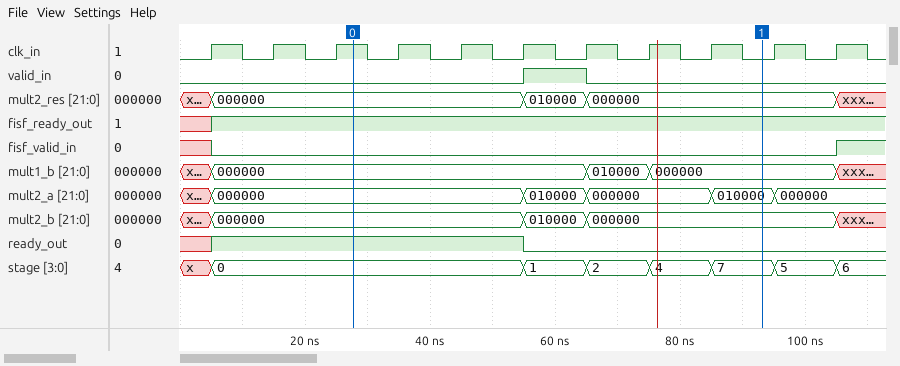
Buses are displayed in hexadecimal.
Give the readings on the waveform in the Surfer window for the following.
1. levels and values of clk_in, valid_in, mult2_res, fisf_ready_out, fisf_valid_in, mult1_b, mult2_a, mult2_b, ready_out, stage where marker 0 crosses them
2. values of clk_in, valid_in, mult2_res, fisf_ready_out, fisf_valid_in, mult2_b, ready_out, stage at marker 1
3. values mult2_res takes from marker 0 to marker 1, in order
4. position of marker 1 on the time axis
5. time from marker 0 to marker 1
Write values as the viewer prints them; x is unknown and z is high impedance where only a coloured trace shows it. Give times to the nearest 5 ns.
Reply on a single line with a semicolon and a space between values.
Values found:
clk_in=1, valid_in=0, mult2_res=000000, fisf_ready_out=1, fisf_valid_in=0, mult1_b=000000, mult2_a=000000, mult2_b=000000, ready_out=1, stage=0; clk_in=0, valid_in=0, mult2_res=000000, fisf_ready_out=1, fisf_valid_in=0, mult2_b=000000, ready_out=0, stage=7; 000000, 010000, 000000; 95 ns; 65 ns
